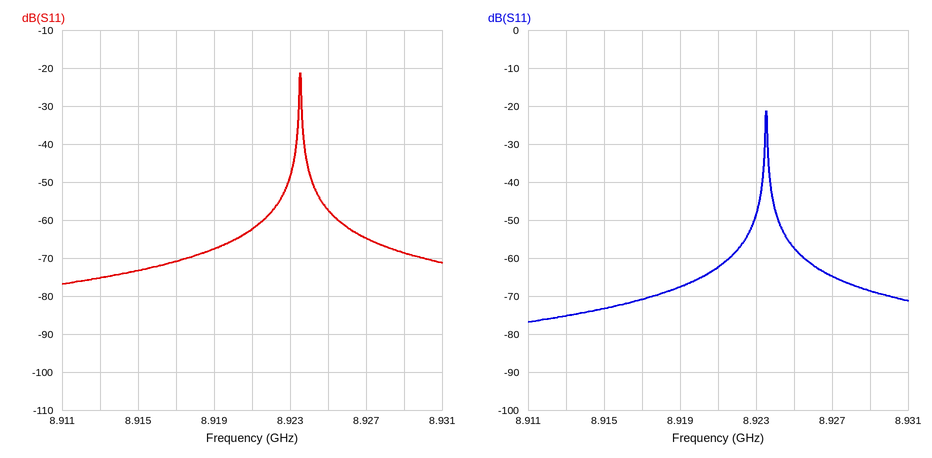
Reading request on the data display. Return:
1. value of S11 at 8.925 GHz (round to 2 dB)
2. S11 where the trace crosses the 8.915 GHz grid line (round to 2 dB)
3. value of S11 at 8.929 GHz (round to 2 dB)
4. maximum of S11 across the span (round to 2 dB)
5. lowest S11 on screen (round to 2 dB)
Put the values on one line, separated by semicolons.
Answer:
-58 dB; -74 dB; -68 dB; -22 dB; -76 dB
